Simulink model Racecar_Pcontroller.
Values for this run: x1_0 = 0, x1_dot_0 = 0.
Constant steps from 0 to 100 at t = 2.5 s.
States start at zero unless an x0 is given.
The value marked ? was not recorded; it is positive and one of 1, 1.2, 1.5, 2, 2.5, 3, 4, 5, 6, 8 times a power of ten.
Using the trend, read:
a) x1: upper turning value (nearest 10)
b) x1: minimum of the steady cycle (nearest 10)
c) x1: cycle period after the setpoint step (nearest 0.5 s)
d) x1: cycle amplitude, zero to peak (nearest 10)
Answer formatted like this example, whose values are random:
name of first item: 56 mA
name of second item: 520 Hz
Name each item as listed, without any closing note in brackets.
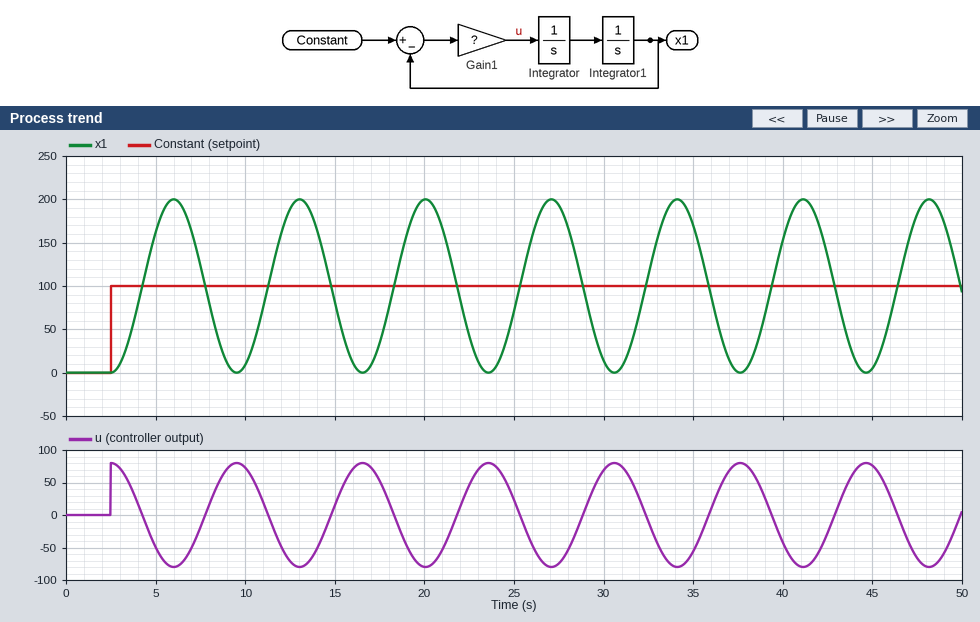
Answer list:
x1: upper turning value: 200
x1: minimum of the steady cycle: 0
x1: cycle period after the setpoint step: 7.0 s
x1: cycle amplitude, zero to peak: 100
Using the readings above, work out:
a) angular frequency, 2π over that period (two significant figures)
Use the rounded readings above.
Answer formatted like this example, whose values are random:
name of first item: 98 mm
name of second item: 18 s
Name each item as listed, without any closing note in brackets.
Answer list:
angular frequency, 2π over that period: 0.90 rad/s
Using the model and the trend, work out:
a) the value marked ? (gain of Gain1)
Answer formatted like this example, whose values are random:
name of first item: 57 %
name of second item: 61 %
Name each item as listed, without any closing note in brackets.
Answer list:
the value marked ?: 0.8
